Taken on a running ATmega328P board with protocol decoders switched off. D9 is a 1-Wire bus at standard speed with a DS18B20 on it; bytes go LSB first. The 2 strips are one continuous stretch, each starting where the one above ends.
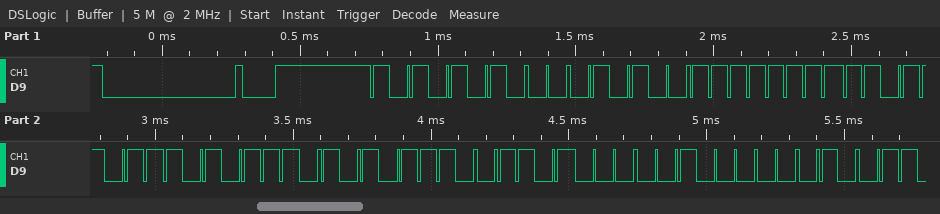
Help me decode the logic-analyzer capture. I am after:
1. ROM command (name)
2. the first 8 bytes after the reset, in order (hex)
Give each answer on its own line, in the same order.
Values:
Match ROM
55 28 FF DB 75 75 16 04
